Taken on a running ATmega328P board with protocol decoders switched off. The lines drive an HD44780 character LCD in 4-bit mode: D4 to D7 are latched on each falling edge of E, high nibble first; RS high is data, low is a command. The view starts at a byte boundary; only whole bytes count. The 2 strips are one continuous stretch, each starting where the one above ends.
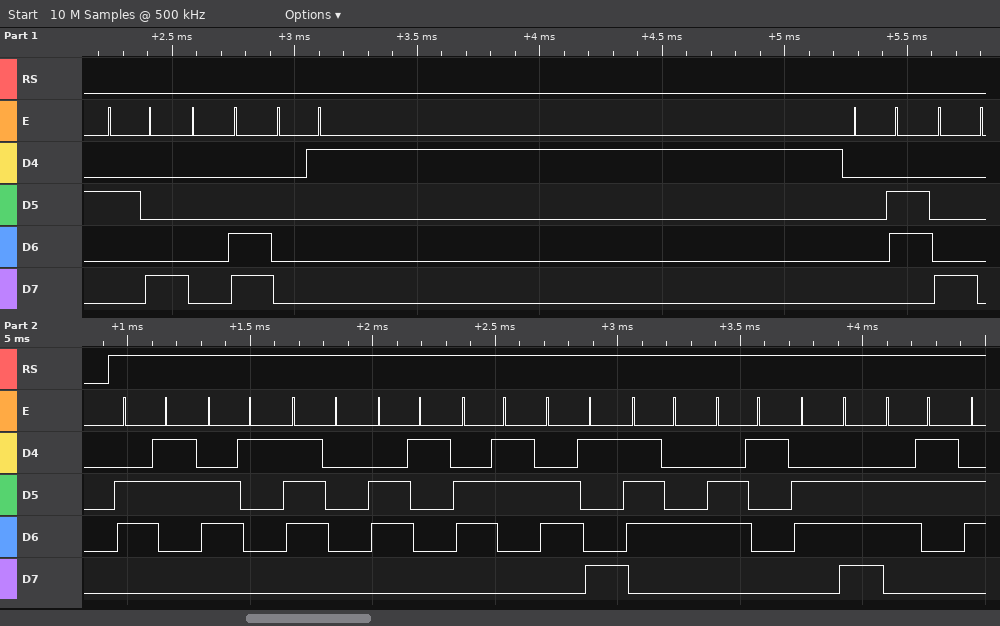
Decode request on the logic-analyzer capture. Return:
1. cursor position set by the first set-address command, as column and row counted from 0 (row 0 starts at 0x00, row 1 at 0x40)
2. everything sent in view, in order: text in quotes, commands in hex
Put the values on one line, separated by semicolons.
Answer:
column 0, row 0; 0x28 0x0C 0x01 0x06 0x80 "capacitanc"
